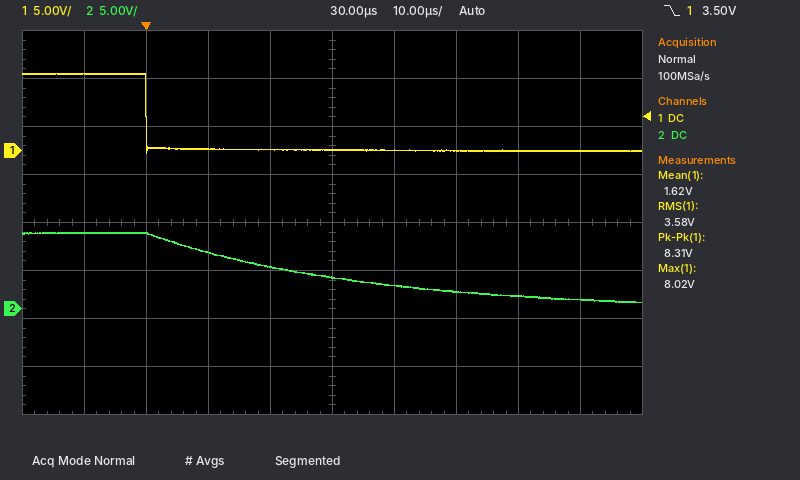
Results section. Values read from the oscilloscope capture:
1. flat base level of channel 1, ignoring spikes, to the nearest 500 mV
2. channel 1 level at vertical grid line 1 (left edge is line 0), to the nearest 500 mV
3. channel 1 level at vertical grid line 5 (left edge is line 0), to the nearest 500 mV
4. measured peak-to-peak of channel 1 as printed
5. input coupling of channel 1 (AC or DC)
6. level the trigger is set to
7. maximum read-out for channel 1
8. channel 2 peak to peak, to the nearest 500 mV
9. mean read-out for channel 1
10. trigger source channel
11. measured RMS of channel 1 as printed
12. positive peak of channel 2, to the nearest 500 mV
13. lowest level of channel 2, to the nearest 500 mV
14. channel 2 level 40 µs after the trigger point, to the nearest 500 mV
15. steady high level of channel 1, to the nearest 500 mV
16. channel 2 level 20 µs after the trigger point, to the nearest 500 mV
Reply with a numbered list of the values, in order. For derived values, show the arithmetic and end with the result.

1. 0.0 V
2. 8.0 V
3. 0.0 V
4. 8.31 V
5. DC
6. 3.50 V
7. 8.02 V
8. 8.0 V − (500 mV) = 7.5 V
9. 1.62 V
10. channel 1
11. 3.58 V
12. 8.0 V
13. 500 mV
14. 2.5 V
15. 8.0 V
16. 4.5 V
